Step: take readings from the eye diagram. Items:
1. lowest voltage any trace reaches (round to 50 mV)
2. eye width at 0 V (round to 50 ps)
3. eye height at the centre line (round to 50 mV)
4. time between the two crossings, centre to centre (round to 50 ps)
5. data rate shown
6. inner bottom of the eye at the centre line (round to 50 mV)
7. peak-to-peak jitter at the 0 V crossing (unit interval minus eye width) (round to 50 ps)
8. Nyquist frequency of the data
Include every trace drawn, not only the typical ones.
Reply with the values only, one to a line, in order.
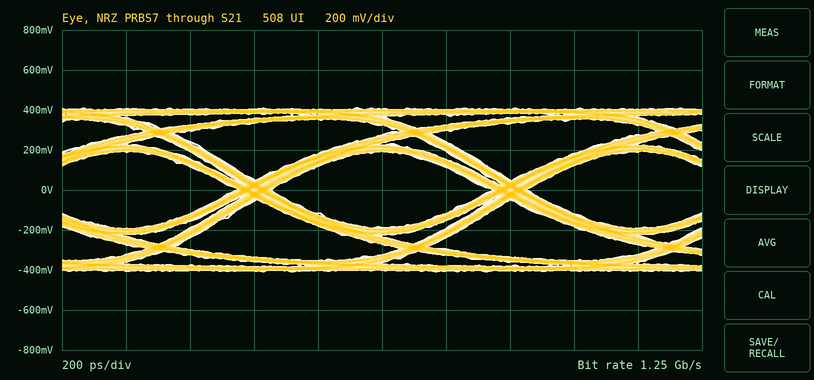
-400 mV
700 ps
400 mV
800 ps
1.25 Gb/s
-200 mV
100 ps
625 MHz
